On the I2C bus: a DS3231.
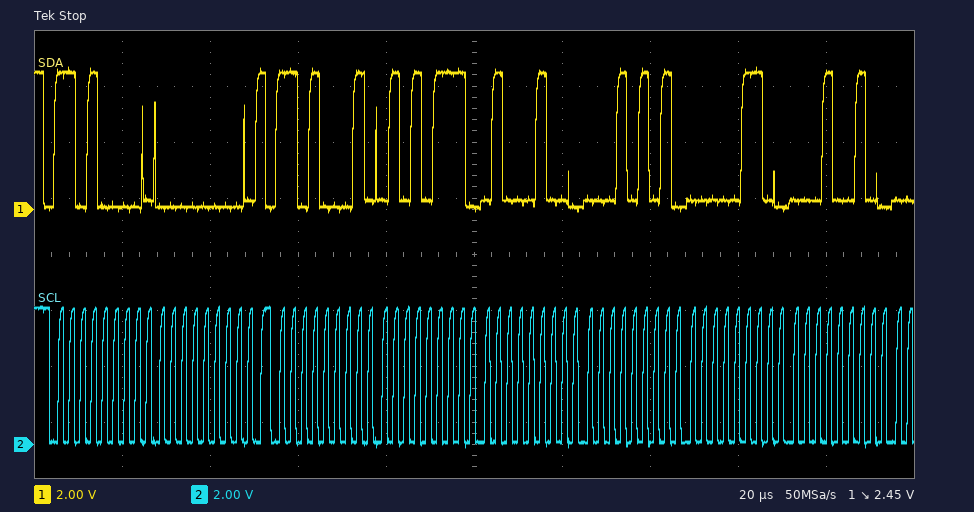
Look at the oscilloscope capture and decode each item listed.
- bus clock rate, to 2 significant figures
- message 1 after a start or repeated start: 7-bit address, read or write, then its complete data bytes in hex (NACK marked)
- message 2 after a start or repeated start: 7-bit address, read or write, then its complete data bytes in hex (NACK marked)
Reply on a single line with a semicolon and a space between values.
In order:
400 kHz; 0x68 write: 00; 0x68 read: 57 44 15 06 12
